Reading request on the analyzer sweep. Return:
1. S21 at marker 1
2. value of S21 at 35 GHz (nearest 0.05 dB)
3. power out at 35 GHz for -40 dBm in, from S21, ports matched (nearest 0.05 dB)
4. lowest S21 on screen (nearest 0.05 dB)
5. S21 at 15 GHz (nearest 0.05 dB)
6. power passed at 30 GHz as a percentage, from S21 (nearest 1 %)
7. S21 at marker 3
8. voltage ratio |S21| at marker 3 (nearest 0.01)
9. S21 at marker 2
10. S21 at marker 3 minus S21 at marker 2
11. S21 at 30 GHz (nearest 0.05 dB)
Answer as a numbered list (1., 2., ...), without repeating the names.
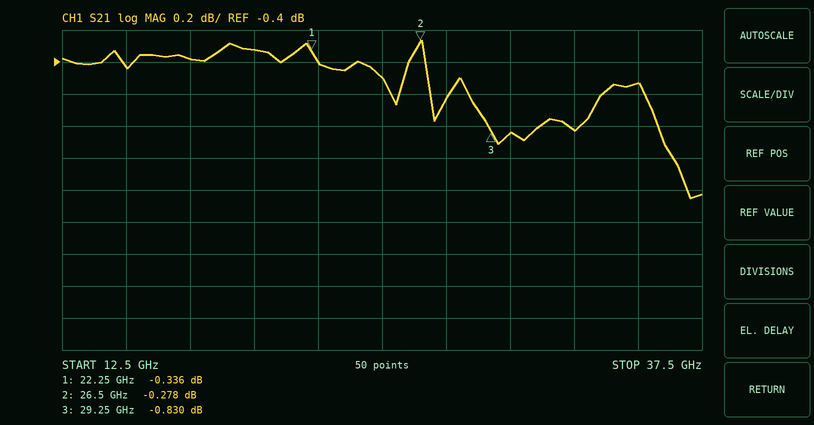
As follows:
1. -0.336 dB
2. -0.55 dB
3. -40.55 dBm
4. -1.25 dB
5. -0.45 dB
6. 82 %
7. -0.830 dB
8. 0.91
9. -0.278 dB
10. -0.552 dB
11. -0.85 dB
